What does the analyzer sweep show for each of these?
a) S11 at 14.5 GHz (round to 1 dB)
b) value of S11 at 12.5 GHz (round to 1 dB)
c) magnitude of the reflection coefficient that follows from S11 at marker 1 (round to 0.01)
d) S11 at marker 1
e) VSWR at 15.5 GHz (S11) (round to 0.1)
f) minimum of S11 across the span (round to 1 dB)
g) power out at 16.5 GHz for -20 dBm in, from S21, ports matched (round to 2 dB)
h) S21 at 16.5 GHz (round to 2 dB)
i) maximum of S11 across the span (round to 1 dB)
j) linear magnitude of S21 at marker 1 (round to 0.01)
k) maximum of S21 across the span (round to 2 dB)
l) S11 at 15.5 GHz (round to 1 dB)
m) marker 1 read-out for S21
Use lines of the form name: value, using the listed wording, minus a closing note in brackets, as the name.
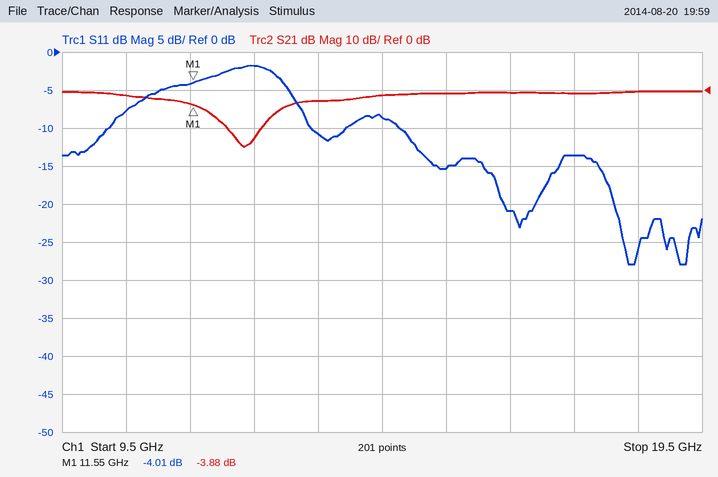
S11 at 14.5 GHz: -9 dB
value of S11 at 12.5 GHz: -2 dB
magnitude of the reflection coefficient that follows from S11 at marker 1: 0.63
S11 at marker 1: -4.01 dB
VSWR at 15.5 GHz (S11): 1.4
minimum of S11 across the span: -28 dB
power out at 16.5 GHz for -20 dBm in, from S21, ports matched: -20 dBm
S21 at 16.5 GHz: 0 dB
maximum of S11 across the span: -2 dB
linear magnitude of S21 at marker 1: 0.64
maximum of S21 across the span: 0 dB
S11 at 15.5 GHz: -15 dB
marker 1 read-out for S21: -3.88 dB
